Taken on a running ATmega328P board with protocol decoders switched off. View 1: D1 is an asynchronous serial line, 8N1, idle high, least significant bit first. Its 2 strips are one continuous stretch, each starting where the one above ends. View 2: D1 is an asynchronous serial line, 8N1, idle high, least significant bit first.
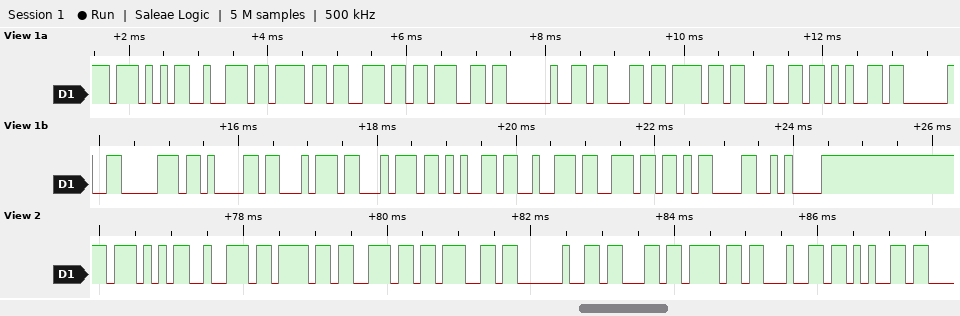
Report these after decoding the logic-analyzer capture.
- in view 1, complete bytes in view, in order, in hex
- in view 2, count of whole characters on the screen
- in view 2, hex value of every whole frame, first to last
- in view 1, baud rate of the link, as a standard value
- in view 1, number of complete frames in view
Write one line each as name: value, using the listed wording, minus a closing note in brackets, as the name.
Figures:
in view 1, complete bytes in view, in order, in hex: 57 72 6F 6E 67 20 63 6F 64 65 20 70 61 74 74 65 72 6E 0D 0A
in view 2, count of whole characters on the screen: 10
in view 2, hex value of every whole frame, first to last: 0x57 0x72 0x6F 0x6E 0x67 0x20 0x63 0x6F 0x64 0x65
in view 1, baud rate of the link, as a standard value: 9600 baud
in view 1, number of complete frames in view: 20
